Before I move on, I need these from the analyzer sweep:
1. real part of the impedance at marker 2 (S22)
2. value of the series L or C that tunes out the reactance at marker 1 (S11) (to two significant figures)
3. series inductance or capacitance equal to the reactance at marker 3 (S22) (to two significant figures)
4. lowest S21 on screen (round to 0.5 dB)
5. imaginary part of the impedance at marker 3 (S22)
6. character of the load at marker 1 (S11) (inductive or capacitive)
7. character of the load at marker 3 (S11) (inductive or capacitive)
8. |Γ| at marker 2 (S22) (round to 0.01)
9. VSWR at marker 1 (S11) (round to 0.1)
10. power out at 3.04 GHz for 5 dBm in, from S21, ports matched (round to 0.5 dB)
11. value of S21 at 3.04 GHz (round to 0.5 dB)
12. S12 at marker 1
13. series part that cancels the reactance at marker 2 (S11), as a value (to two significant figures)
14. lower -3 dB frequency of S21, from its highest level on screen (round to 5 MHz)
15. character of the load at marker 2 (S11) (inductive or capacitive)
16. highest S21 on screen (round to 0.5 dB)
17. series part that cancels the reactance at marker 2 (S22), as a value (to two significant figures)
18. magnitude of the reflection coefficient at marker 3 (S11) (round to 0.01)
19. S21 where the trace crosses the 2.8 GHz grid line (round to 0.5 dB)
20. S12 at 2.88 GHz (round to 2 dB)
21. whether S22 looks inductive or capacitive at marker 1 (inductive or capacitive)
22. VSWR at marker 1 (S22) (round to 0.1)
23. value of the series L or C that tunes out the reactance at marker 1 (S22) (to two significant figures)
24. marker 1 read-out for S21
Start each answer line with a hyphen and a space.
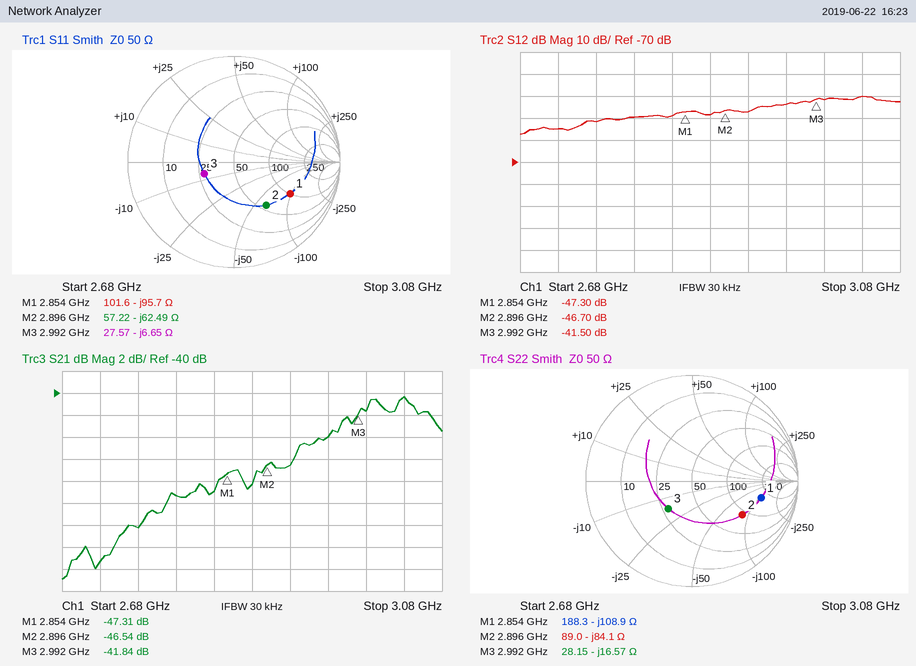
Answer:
- 89.0 Ω
- 5.3 nH
- 3.2 pF
- -57.0 dB
- -16.57 Ω
- capacitive
- capacitive
- 0.57
- 4.1
- -35.5 dBm
- -40.5 dB
- -47.30 dB
- 3.4 nH
- 2.970 GHz
- capacitive
- -40.5 dB
- 4.6 nH
- 0.30
- -49.5 dB
- -48 dB
- capacitive
- 5.1
- 6.1 nH
- -47.31 dB
